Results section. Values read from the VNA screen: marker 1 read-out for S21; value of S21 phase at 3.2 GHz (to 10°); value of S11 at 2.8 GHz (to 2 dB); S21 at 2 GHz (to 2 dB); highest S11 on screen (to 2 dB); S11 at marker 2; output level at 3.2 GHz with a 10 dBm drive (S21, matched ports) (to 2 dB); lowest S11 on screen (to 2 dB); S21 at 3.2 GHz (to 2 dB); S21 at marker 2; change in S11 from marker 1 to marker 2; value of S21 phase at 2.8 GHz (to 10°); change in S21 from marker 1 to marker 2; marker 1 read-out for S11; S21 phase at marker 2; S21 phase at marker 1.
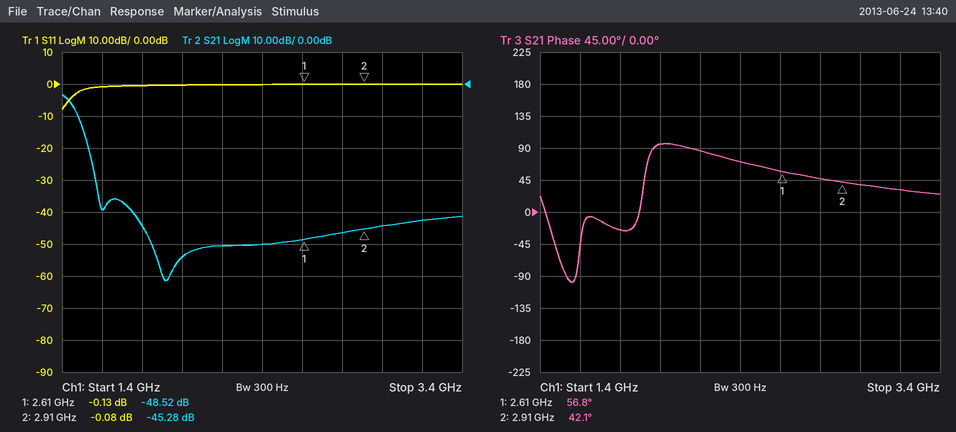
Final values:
-48.52 dB
30°
0 dB
-54 dB
0 dB
-0.08 dB
-32 dBm
-8 dB
-42 dB
-45.28 dB
0.05 dB
50°
3.24 dB
-0.13 dB
42.1°
56.8°
